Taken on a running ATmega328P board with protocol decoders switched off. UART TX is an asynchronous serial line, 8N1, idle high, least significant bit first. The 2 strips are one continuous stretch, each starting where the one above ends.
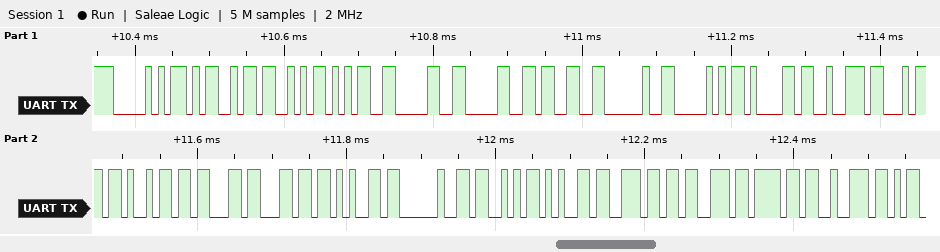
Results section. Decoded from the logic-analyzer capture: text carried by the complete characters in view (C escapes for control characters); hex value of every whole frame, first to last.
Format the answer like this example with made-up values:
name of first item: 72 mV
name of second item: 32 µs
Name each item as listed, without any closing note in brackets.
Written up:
text carried by the complete characters in view: "PMS5003 Particle Sensor"
hex value of every whole frame, first to last: 50 4D 53 35 30 30 33 20 50 61 72 74 69 63 6C 65 20 53 65 6E 73 6F 72
